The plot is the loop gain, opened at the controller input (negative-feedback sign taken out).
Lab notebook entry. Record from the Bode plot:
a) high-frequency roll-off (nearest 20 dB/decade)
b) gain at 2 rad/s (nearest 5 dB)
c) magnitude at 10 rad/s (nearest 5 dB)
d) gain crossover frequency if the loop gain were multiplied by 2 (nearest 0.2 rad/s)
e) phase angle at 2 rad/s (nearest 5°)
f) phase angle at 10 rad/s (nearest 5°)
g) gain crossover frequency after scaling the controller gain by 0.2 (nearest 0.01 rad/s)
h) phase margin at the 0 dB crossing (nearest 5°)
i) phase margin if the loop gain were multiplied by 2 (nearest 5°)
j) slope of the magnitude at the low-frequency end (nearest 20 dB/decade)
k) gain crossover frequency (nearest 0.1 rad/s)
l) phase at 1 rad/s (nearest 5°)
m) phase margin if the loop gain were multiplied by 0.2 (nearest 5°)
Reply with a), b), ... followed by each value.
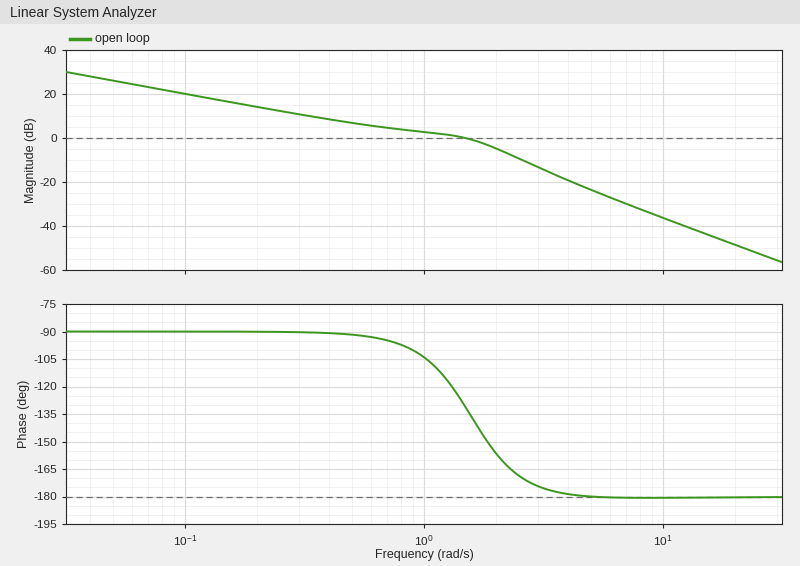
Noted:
a) -40 dB/decade
b) -5 dB
c) -35 dB
d) 2.2 rad/s
e) -155°
f) -180°
g) 0.20 rad/s
h) 50°
i) 20°
j) -20 dB/decade
k) 1.5 rad/s
l) -105°
m) 90°
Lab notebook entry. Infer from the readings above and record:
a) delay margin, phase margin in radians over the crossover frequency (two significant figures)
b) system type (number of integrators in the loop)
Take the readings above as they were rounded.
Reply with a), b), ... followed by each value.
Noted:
a) 0.58 s
b) 1
